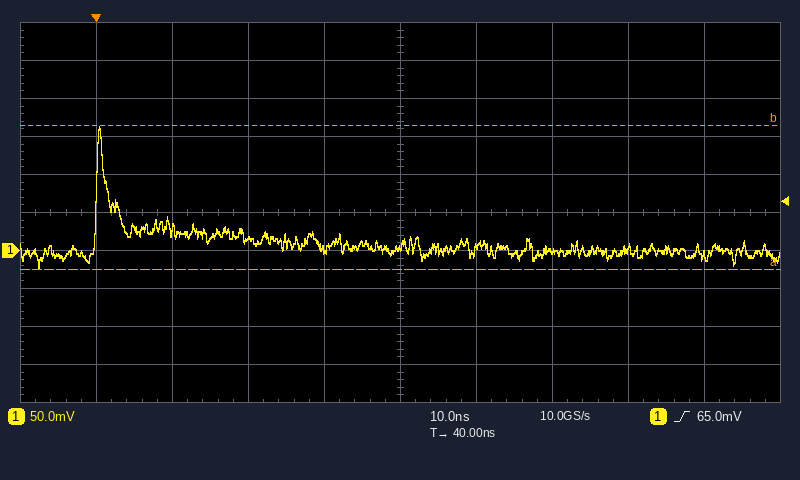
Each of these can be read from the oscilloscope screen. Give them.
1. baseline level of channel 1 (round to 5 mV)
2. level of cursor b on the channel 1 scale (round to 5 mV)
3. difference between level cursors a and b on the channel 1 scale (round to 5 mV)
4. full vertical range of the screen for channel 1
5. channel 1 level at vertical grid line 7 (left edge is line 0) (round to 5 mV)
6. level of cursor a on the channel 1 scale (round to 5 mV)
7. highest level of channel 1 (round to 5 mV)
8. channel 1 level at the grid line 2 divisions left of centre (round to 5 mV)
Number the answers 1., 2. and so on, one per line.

1. 0 mV
2. 165 mV
3. 190 mV
4. 500 mV
5. 0 mV
6. -25 mV
7. 165 mV
8. 15 mV
